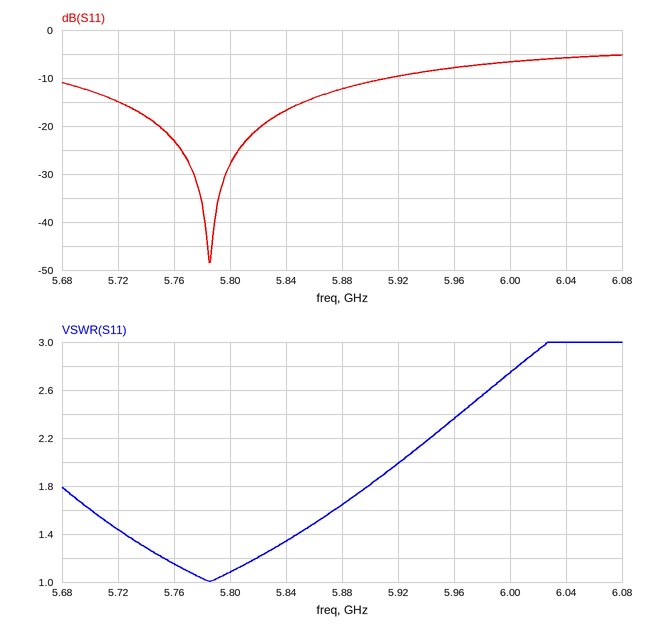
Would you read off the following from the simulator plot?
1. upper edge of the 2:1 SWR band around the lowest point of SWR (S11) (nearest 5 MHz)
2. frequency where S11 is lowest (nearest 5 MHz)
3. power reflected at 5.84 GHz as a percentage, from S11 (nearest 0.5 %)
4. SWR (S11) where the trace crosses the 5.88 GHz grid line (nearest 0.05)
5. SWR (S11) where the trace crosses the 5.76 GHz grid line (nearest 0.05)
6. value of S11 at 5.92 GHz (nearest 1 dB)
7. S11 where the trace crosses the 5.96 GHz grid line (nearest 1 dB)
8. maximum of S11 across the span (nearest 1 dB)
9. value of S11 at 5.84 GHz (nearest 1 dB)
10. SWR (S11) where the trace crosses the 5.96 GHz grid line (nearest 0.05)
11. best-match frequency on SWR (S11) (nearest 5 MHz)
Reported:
5.920 GHz
5.785 GHz
2.0 %
1.65
1.15
-10 dB
-8 dB
-5 dB
-17 dB
2.35
5.785 GHz
